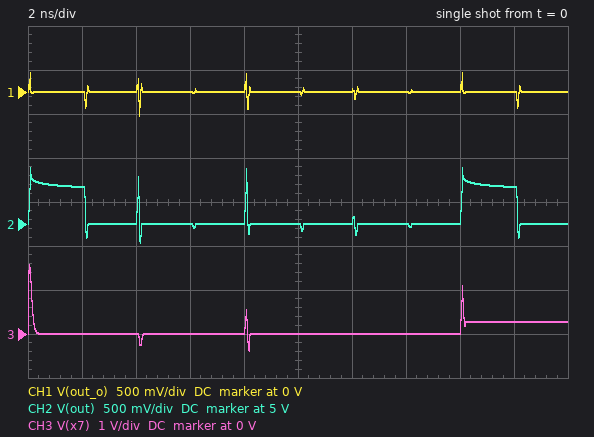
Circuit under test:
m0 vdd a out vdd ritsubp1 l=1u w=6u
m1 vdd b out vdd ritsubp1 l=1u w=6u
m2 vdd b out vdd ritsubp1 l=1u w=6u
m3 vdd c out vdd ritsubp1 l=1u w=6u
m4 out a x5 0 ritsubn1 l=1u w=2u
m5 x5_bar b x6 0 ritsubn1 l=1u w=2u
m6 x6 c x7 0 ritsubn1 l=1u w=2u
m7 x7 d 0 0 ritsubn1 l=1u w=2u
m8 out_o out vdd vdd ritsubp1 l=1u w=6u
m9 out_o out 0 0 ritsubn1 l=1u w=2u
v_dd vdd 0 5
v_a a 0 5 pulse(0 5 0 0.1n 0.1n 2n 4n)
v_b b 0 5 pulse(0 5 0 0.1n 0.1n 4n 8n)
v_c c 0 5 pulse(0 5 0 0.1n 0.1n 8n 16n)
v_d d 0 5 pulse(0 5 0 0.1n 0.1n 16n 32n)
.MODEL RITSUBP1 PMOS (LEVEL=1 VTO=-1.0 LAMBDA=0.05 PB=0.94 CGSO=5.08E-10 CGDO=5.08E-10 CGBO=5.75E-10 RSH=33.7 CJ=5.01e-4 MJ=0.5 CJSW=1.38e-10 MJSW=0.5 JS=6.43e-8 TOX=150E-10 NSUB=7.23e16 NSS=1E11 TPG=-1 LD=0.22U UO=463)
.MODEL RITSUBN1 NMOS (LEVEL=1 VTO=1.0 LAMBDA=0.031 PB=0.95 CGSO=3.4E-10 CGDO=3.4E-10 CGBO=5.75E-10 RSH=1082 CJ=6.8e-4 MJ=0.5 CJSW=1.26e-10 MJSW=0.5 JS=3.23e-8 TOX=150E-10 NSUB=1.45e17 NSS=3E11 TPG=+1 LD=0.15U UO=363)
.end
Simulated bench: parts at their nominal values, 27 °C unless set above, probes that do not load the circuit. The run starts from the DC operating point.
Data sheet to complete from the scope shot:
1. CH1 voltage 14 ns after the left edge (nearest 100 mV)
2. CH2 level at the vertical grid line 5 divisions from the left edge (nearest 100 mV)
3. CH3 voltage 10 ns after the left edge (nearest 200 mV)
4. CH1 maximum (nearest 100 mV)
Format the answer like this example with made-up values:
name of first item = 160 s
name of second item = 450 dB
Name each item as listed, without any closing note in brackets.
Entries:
CH1 voltage 14 ns after the left edge = 0 V
CH2 level at the vertical grid line 5 divisions from the left edge = 5.0 V
CH3 voltage 10 ns after the left edge = 0 V
CH1 maximum = 200 mV
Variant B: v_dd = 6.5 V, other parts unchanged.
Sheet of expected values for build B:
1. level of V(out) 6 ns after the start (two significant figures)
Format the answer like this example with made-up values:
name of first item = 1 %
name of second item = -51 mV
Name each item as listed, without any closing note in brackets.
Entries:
level of V(out) 6 ns after the start = 6.5 V
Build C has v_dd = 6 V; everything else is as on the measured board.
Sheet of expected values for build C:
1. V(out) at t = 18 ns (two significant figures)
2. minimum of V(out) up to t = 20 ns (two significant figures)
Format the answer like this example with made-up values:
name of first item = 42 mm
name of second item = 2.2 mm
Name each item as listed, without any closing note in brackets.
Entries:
V(out) at t = 18 ns = 6.0 V
minimum of V(out) up to t = 20 ns = 5.8 V
